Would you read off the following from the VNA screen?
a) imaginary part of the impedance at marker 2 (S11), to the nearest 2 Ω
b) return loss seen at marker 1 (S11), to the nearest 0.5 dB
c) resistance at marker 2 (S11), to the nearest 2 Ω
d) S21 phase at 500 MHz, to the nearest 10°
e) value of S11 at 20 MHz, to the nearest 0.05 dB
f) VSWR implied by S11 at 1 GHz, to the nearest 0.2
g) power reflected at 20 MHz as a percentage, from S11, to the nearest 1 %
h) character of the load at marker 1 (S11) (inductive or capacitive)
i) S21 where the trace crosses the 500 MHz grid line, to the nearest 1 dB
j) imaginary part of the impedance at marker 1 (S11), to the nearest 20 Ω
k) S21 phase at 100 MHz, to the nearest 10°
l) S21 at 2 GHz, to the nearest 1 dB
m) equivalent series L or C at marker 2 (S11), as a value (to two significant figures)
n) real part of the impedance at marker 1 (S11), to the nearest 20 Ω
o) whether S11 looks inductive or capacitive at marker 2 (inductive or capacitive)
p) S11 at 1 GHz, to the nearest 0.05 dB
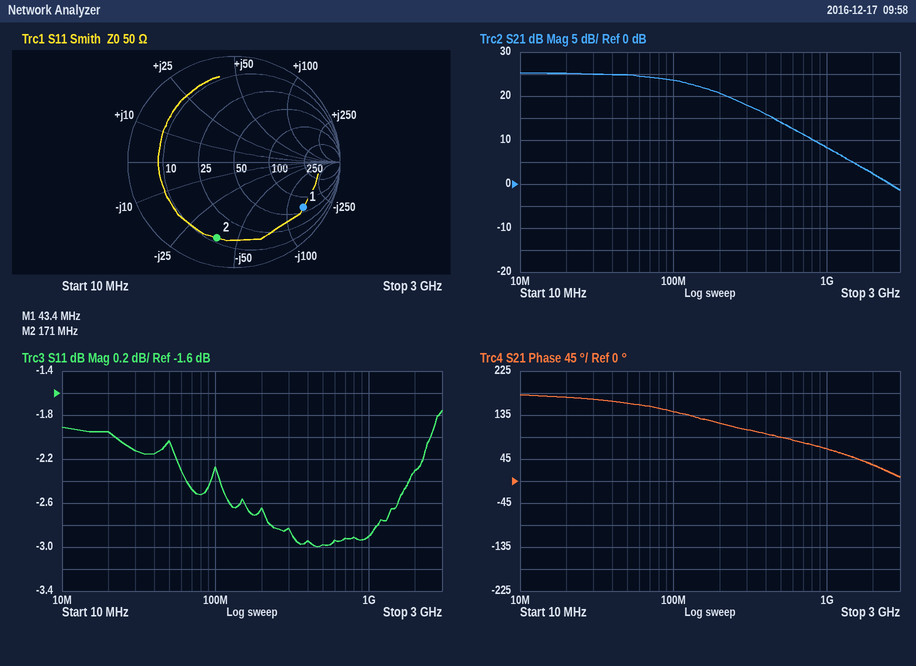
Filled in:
-38 Ω
2.0 dB
12 Ω
90°
-1.95 dB
6.0
64 %
capacitive
14 dB
-140 Ω
140°
2 dB
24 pF
60 Ω
capacitive
-2.90 dB
